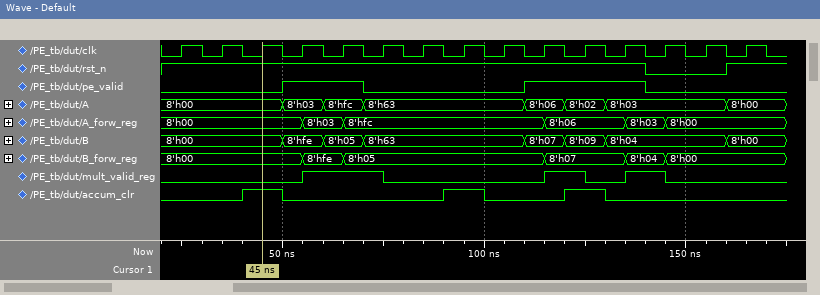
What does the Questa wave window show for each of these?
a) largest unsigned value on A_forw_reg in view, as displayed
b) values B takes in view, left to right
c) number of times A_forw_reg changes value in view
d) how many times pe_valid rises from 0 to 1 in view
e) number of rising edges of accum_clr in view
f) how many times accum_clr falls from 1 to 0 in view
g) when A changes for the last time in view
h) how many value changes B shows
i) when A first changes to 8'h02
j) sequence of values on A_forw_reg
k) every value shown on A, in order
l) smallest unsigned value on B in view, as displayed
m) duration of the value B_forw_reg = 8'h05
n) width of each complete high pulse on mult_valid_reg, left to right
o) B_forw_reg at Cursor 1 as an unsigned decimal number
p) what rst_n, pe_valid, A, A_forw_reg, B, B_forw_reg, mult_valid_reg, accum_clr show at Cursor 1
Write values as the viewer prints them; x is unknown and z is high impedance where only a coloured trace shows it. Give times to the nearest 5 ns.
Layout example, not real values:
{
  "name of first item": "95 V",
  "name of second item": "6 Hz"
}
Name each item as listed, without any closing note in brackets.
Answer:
{
  "largest unsigned value on A_forw_reg in view, as displayed": "8'hfc",
  "values B takes in view, left to right": "8'h00, 8'hfe, 8'h05, 8'h63, 8'h07, 8'h09, 8'h04, 8'h00",
  "number of times A_forw_reg changes value in view": "5",
  "how many times pe_valid rises from 0 to 1 in view": "2",
  "number of rising edges of accum_clr in view": "3",
  "how many times accum_clr falls from 1 to 0 in view": "3",
  "when A changes for the last time in view": "160 ns",
  "how many value changes B shows": "7",
  "when A first changes to 8'h02": "120 ns",
  "sequence of values on A_forw_reg": "8'h00, 8'h03, 8'hfc, 8'h06, 8'h03, 8'h00",
  "every value shown on A, in order": "8'h00, 8'h03, 8'hfc, 8'h63, 8'h06, 8'h02, 8'h03, 8'h00",
  "smallest unsigned value on B in view, as displayed": "8'h00",
  "duration of the value B_forw_reg = 8'h05": "50 ns",
  "width of each complete high pulse on mult_valid_reg, left to right": "20 ns, 10 ns, 10 ns",
  "B_forw_reg at Cursor 1 as an unsigned decimal number": "0",
  "what rst_n, pe_valid, A, A_forw_reg, B, B_forw_reg, mult_valid_reg, accum_clr show at Cursor 1": "rst_n=1, pe_valid=0, A=8'h00, A_forw_reg=8'h00, B=8'h00, B_forw_reg=8'h00, mult_valid_reg=0, accum_clr=1"
}
